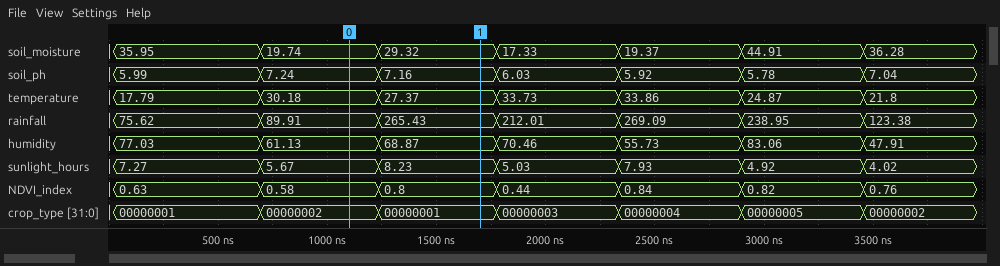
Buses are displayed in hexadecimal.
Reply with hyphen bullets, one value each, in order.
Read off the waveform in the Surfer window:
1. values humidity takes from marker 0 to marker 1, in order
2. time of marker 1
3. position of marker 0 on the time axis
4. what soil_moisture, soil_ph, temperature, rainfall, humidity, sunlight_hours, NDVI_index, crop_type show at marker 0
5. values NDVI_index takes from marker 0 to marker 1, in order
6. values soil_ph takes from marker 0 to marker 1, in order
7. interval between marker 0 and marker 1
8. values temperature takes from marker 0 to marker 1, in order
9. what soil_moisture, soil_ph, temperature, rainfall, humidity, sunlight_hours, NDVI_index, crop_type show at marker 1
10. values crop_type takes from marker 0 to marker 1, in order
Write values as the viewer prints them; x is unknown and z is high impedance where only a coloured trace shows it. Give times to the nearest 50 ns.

- 61.13, 68.87
- 1700 ns
- 1100 ns
- soil_moisture=19.74, soil_ph=7.24, temperature=30.18, rainfall=89.91, humidity=61.13, sunlight_hours=5.67, NDVI_index=0.58, crop_type=00000002
- 0.58, 0.8
- 7.24, 7.16
- 600 ns
- 30.18, 27.37
- soil_moisture=29.32, soil_ph=7.16, temperature=27.37, rainfall=265.43, humidity=68.87, sunlight_hours=8.23, NDVI_index=0.8, crop_type=00000001
- 00000002, 00000001
